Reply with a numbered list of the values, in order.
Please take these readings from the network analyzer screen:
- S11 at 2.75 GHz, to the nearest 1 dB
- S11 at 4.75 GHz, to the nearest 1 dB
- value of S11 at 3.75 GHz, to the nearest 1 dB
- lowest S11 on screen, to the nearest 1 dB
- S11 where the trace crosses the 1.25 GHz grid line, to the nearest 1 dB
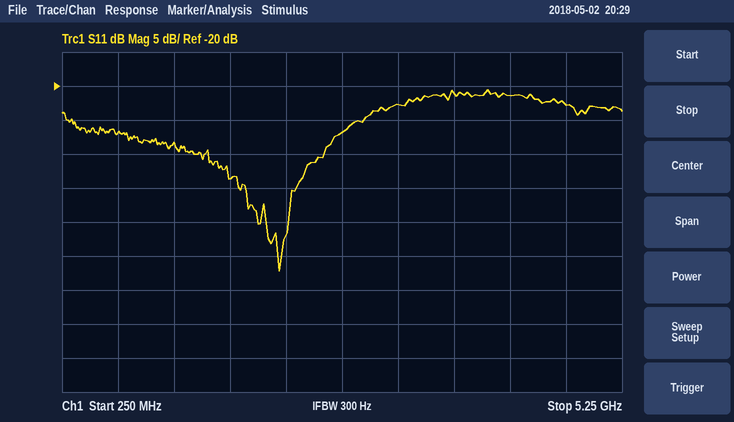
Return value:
1. -27 dB
2. -23 dB
3. -21 dB
4. -47 dB
5. -28 dB
